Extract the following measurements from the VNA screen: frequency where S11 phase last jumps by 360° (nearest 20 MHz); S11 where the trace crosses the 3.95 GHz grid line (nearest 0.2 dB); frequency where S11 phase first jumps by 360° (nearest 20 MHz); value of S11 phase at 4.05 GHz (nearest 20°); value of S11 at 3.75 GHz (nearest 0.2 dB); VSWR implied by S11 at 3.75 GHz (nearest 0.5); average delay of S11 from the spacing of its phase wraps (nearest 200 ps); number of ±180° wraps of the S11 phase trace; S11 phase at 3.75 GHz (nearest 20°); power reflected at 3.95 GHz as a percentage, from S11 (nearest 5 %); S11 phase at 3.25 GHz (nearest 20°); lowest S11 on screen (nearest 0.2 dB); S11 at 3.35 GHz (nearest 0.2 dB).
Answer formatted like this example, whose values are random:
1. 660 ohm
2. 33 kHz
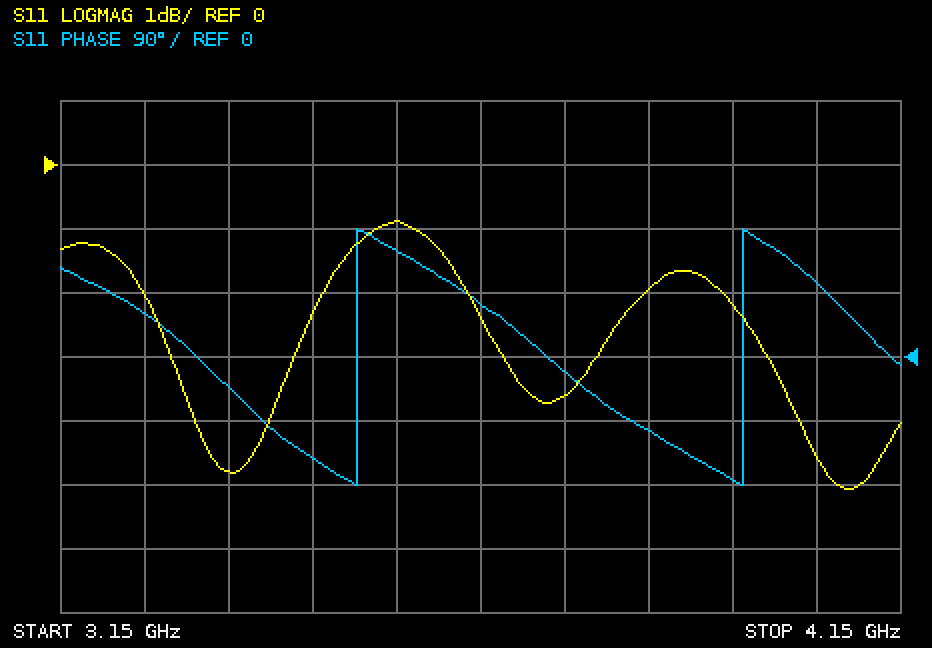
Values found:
1. 3.96 GHz
2. -2.2 dB
3. 3.50 GHz
4. 100°
5. -3.6 dB
6. 5.0
7. 2.2 ns
8. 2
9. -20°
10. 60 %
11. 60°
12. -5.0 dB
13. -4.8 dB
